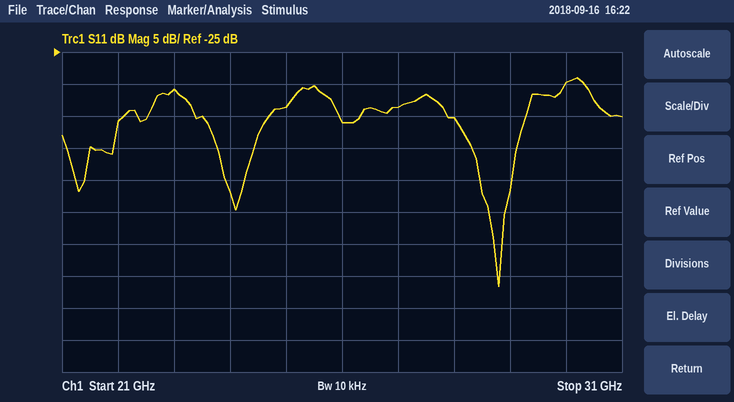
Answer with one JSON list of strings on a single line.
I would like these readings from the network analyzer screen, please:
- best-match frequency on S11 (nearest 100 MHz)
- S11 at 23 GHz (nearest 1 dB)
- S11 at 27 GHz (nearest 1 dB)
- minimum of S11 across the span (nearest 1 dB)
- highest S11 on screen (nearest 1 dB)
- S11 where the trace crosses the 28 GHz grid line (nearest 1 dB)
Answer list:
["28.8 GHz", "-31 dB", "-34 dB", "-62 dB", "-29 dB", "-35 dB"]
